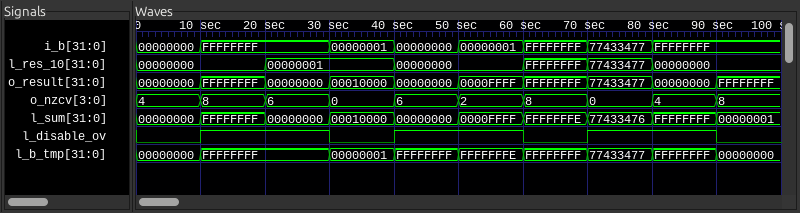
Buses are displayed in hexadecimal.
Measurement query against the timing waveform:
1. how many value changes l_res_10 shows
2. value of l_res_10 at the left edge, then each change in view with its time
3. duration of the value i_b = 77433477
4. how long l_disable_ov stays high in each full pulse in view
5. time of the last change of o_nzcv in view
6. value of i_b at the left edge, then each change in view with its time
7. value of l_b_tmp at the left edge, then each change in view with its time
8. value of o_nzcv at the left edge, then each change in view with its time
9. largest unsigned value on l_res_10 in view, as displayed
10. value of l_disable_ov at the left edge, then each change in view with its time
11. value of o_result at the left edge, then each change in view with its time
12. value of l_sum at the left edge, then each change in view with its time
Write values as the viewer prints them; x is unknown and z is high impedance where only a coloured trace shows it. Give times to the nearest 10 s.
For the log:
5
00000000, 00000001 at 20 s, 00000000 at 40 s, FFFFFFFF at 60 s, 77433477 at 70 s, 00000000 at 80 s
10 s
20 s, 20 s, 20 s
90 s
00000000, FFFFFFFF at 10 s, 00000001 at 30 s, 00000000 at 40 s, 00000001 at 50 s, FFFFFFFF at 60 s, 77433477 at 70 s, FFFFFFFF at 80 s
00000000, FFFFFFFF at 10 s, 00000001 at 30 s, FFFFFFFF at 40 s, FFFFFFFE at 50 s, FFFFFFFF at 60 s, 77433477 at 70 s, FFFFFFFF at 80 s, 00000000 at 90 s
4, 8 at 10 s, 6 at 20 s, 0 at 30 s, 6 at 40 s, 2 at 50 s, 8 at 60 s, 0 at 70 s, 4 at 80 s, 8 at 90 s
FFFFFFFF
0, 1 at 10 s, 0 at 30 s, 1 at 40 s, 0 at 60 s, 1 at 70 s, 0 at 90 s
00000000, FFFFFFFF at 10 s, 00000000 at 20 s, 00010000 at 30 s, 00000000 at 40 s, 0000FFFF at 50 s, FFFFFFFF at 60 s, 77433477 at 70 s, 00000000 at 80 s, FFFFFFFF at 90 s
00000000, FFFFFFFF at 10 s, 00000000 at 20 s, 00010000 at 30 s, 00000000 at 40 s, 0000FFFF at 50 s, FFFFFFFE at 60 s, 77433476 at 70 s, FFFFFFFF at 80 s, 00000001 at 90 s
